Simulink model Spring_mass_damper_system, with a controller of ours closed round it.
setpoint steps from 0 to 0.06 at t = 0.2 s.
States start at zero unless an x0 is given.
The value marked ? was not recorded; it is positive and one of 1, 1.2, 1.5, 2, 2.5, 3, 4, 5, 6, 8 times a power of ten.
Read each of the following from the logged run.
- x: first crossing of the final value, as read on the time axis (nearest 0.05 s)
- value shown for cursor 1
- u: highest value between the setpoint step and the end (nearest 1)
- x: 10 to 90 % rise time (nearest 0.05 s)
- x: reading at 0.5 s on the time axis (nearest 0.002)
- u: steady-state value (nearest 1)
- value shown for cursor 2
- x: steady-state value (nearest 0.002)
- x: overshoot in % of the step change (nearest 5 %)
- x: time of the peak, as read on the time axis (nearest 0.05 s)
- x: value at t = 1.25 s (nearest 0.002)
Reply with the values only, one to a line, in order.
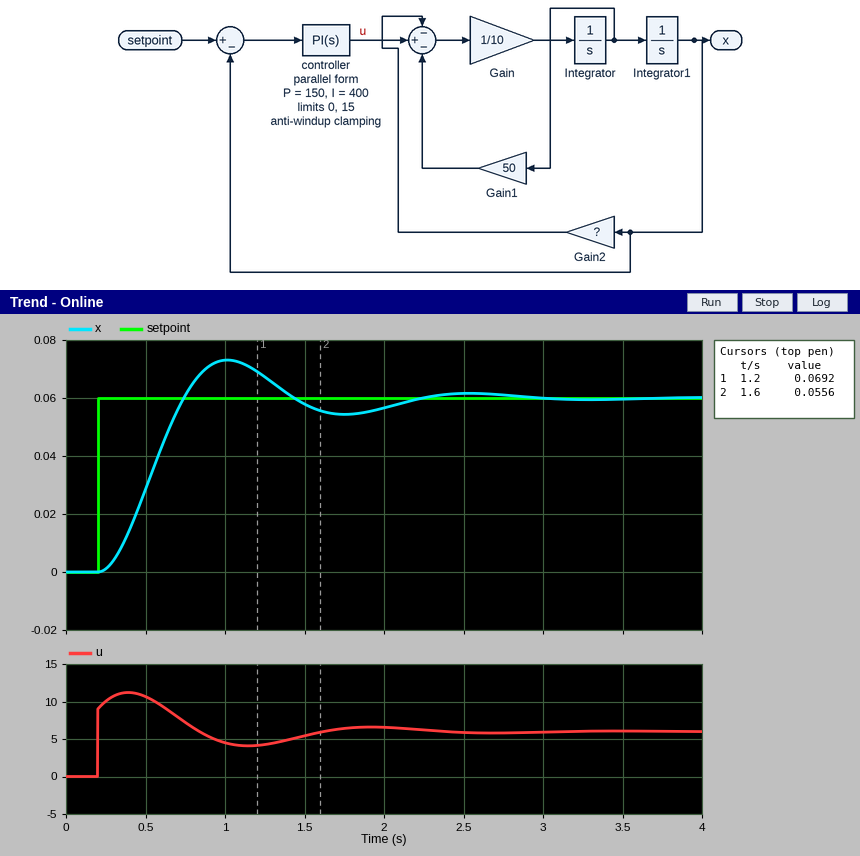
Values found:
0.75 s
0.0692
11
0.35 s
0.028
6
0.0556
0.060
20 %
1.00 s
0.068
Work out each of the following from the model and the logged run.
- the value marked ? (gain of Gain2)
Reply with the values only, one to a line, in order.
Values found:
100
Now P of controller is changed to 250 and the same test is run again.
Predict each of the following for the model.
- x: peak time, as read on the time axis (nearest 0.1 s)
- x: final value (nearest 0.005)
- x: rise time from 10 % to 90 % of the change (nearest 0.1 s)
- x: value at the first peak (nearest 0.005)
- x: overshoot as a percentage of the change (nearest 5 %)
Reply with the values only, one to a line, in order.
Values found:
0.8 s
0.060
0.3 s
0.070
15 %
